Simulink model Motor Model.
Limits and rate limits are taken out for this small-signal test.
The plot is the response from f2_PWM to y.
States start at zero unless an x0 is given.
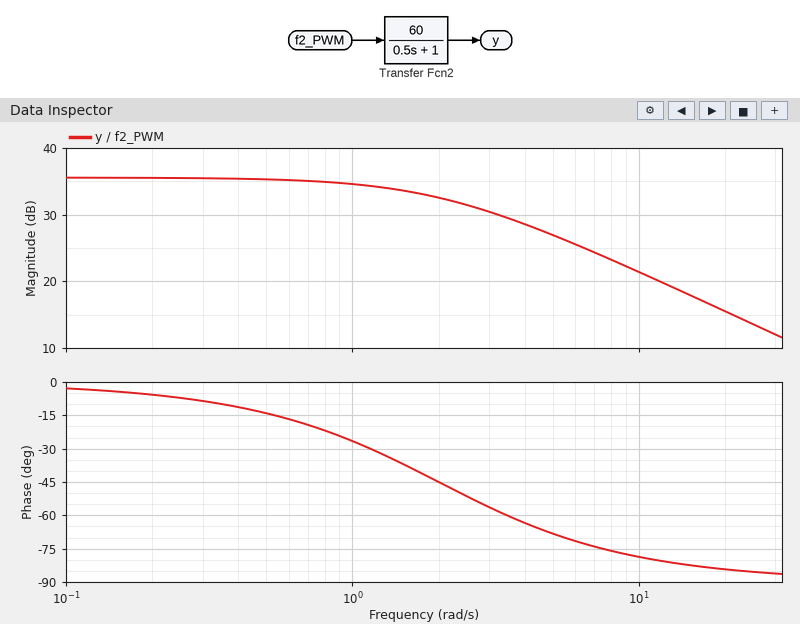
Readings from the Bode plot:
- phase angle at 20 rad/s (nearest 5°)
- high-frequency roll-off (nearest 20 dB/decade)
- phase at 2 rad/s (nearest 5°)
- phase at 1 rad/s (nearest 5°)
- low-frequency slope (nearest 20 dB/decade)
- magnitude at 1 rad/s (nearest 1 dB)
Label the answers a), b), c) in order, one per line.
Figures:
a) -85°
b) -20 dB/decade
c) -45°
d) -25°
e) 0 dB/decade
f) 35 dB
